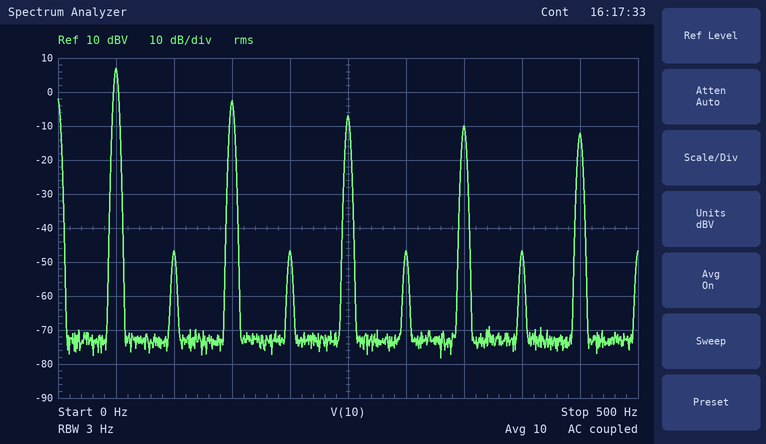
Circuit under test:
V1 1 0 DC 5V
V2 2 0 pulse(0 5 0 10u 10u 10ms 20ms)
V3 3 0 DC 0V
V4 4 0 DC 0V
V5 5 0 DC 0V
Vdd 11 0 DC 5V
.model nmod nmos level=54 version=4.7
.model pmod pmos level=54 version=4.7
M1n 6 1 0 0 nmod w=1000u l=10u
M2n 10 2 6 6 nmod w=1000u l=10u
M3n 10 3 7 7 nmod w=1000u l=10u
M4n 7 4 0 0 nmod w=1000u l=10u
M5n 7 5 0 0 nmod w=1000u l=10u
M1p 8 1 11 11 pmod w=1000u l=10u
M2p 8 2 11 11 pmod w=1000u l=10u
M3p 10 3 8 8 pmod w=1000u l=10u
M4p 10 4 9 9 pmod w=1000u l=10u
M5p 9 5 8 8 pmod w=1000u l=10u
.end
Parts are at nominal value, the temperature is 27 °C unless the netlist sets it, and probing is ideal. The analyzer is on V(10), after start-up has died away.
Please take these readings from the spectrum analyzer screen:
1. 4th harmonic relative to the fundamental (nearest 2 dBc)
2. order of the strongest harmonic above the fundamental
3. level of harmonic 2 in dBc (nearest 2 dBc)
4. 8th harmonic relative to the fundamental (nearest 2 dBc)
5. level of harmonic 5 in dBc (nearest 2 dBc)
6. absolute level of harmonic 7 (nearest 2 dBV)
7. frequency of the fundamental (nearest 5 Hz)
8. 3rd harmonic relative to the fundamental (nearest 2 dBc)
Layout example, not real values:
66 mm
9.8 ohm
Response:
-54 dBc
3
-54 dBc
-54 dBc
-14 dBc
-10 dBV
50 Hz
-10 dBc
